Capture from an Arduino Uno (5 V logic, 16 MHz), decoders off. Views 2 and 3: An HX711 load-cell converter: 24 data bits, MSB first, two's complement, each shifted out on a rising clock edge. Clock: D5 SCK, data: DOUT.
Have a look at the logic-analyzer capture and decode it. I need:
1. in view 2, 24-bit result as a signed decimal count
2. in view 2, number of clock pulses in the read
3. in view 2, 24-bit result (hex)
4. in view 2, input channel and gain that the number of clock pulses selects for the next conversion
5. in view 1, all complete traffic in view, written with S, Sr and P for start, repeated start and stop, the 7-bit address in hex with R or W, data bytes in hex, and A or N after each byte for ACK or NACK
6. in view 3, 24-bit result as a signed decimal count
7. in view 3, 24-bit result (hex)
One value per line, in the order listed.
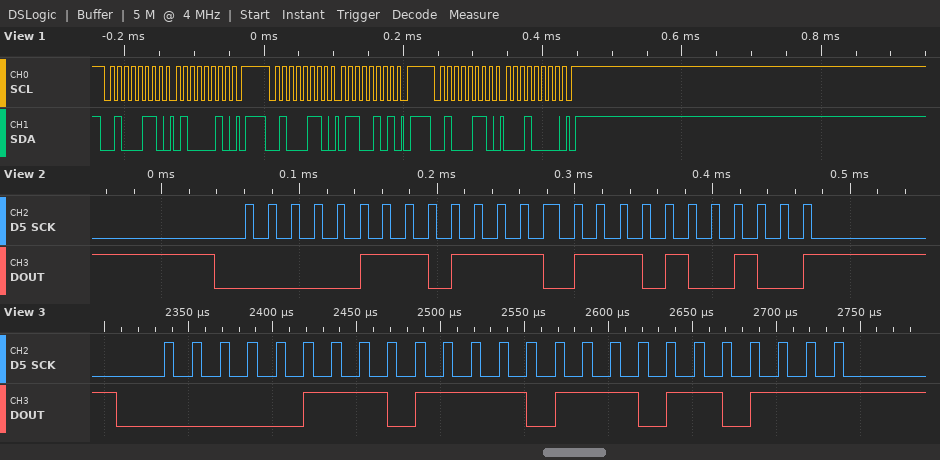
490404
25
0x077BA4
channel A, gain 128
S 23W A 42 A P S 23W A 65 A P S 23W A 10 A P
490423
0x077BB7
